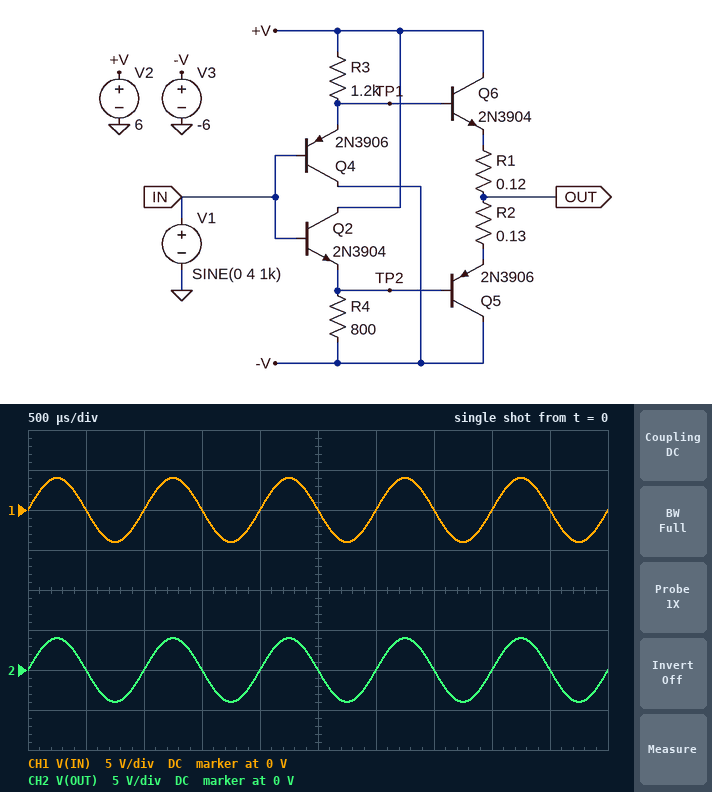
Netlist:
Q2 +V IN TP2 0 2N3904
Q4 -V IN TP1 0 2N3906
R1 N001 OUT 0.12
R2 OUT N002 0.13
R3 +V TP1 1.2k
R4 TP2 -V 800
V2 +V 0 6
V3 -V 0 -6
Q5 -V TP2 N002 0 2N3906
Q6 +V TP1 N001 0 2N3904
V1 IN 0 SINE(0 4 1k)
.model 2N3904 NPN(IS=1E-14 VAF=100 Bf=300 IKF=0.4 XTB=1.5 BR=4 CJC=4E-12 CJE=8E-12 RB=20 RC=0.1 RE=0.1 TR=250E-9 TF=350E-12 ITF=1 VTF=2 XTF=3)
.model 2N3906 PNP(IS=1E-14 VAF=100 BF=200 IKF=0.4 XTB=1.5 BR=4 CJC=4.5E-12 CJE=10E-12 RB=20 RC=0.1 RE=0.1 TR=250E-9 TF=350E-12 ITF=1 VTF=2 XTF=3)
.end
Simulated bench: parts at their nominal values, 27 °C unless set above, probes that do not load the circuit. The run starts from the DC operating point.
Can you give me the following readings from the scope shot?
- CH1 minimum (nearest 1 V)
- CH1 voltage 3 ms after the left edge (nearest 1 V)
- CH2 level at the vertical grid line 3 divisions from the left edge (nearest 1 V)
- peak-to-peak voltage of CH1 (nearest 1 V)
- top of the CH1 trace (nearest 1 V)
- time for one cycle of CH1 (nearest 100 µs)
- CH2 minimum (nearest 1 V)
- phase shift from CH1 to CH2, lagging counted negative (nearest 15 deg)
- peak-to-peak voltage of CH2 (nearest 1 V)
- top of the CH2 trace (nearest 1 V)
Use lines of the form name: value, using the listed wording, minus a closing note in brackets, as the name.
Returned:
CH1 minimum: -4 V
CH1 voltage 3 ms after the left edge: 0 V
CH2 level at the vertical grid line 3 divisions from the left edge: 0 V
peak-to-peak voltage of CH1: 8 V
top of the CH1 trace: 4 V
time for one cycle of CH1: 1.0 ms
CH2 minimum: -4 V
phase shift from CH1 to CH2, lagging counted negative: 0 deg
peak-to-peak voltage of CH2: 8 V
top of the CH2 trace: 4 V
